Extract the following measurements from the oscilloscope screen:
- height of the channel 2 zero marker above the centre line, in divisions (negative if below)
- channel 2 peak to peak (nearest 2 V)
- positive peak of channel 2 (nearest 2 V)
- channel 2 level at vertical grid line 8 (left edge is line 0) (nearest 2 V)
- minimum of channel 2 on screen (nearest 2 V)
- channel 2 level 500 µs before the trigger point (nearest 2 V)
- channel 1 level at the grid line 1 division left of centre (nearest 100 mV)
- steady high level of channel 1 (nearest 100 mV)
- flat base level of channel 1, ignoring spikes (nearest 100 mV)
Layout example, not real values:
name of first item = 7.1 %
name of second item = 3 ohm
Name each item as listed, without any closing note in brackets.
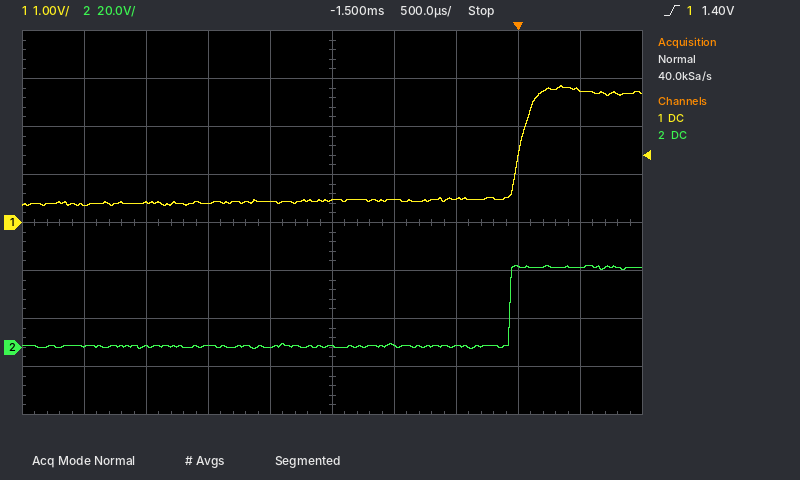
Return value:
height of the channel 2 zero marker above the centre line, in divisions = -2.6 div
channel 2 peak to peak = 34 V
positive peak of channel 2 = 34 V
channel 2 level at vertical grid line 8 (left edge is line 0) = 34 V
minimum of channel 2 on screen = 0 V
channel 2 level 500 µs before the trigger point = 0 V
channel 1 level at the grid line 1 division left of centre = 400 mV
steady high level of channel 1 = 2.7 V
flat base level of channel 1, ignoring spikes = 400 mV
